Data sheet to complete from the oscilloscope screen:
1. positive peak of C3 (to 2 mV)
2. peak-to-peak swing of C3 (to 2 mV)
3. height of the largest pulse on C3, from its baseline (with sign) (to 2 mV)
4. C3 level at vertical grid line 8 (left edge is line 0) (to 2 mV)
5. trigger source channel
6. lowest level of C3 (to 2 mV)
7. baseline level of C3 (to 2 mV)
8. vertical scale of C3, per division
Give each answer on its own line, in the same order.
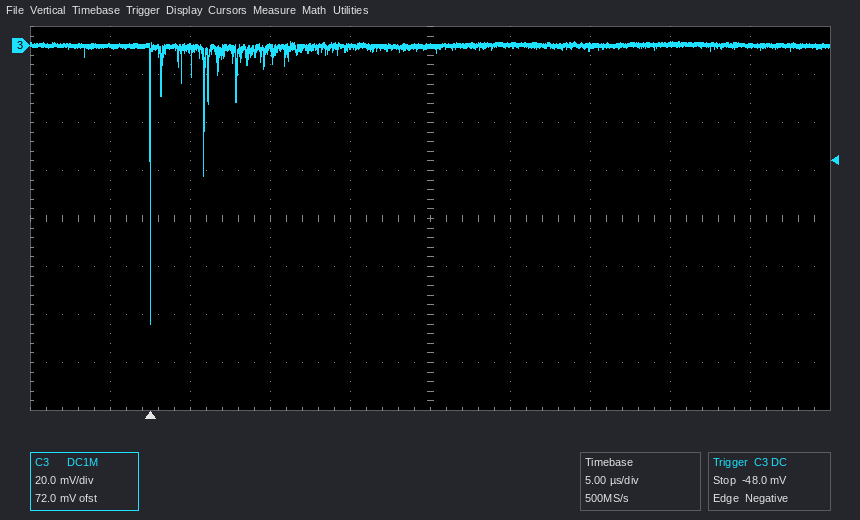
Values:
2 mV
118 mV
-116 mV
0 mV
C3
-116 mV
0 mV
20 mV
